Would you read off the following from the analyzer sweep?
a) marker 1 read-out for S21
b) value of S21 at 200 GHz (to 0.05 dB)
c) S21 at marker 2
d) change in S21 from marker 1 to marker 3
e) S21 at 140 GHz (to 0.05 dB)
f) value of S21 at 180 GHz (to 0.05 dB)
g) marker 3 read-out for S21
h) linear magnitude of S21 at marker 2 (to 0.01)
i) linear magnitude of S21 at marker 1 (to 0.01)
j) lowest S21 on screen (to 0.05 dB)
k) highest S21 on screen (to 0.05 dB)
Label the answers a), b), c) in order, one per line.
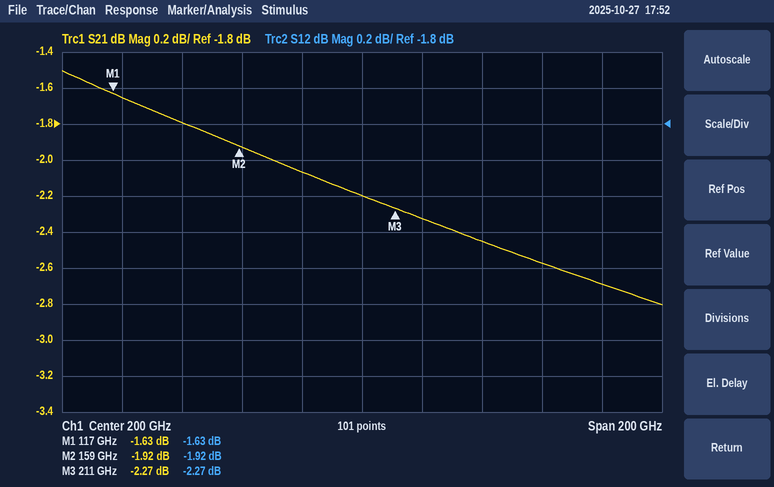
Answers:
a) -1.63 dB
b) -2.20 dB
c) -1.92 dB
d) -0.64 dB
e) -1.80 dB
f) -2.05 dB
g) -2.27 dB
h) 0.80
i) 0.83
j) -2.80 dB
k) -1.50 dB
